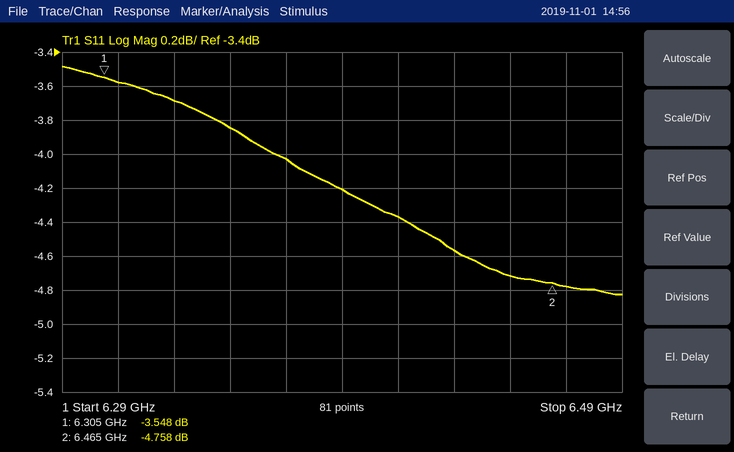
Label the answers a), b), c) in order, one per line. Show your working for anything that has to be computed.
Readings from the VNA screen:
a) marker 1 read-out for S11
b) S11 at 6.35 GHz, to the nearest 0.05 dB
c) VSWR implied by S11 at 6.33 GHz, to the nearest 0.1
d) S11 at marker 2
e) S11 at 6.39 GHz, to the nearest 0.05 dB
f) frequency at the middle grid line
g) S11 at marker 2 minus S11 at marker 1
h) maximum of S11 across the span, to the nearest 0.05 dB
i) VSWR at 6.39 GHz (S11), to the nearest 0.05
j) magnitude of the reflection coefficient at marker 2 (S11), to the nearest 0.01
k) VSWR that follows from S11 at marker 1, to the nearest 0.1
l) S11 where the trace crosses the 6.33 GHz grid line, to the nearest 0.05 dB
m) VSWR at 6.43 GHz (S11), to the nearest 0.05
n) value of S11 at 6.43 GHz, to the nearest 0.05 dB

a) -3.548 dB
b) -3.85 dB
c) |Γ| = 10^(-3.7/20) = 0.6531; VSWR = (1 + 0.6531)/(1 − 0.6531) ≈ 4.8
d) -4.758 dB
e) -4.20 dB
f) 6.39 GHz
g) -4.758 − (-3.548) = -1.210 dB
h) -3.50 dB
i) |Γ| = 10^(-4.2/20) = 0.6166; VSWR = (1 + 0.6166)/(1 − 0.6166) ≈ 4.22, so 4.20 to the nearest 0.05
j) 10^(-4.758/20) ≈ 0.58
k) (1 + 0.6647)/(1 − 0.6647) ≈ 5.0
l) -3.70 dB
m) |Γ| = 10^(-4.55/20) = 0.5922; VSWR = (1 + 0.5922)/(1 − 0.5922) ≈ 3.90
n) -4.55 dB
